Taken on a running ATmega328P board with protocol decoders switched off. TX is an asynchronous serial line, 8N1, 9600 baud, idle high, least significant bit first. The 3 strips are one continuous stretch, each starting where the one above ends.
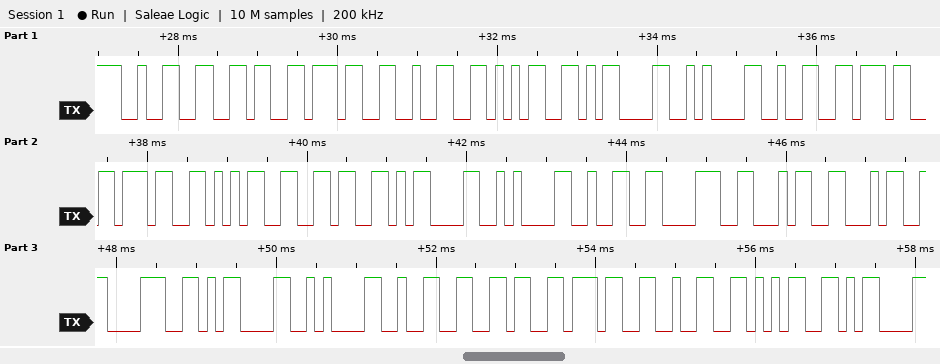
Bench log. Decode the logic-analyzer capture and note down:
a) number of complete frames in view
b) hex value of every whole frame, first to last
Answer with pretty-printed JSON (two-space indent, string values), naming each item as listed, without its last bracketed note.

{
  "number of complete frames in view": "27",
  "hex value of every whole frame, first to last": "32 36 37 32 35 0D 0A 32 37 37 35 36 0D 0A 32 38 34 34 38 0D 0A 32 36 37 32 35 0D"
}
